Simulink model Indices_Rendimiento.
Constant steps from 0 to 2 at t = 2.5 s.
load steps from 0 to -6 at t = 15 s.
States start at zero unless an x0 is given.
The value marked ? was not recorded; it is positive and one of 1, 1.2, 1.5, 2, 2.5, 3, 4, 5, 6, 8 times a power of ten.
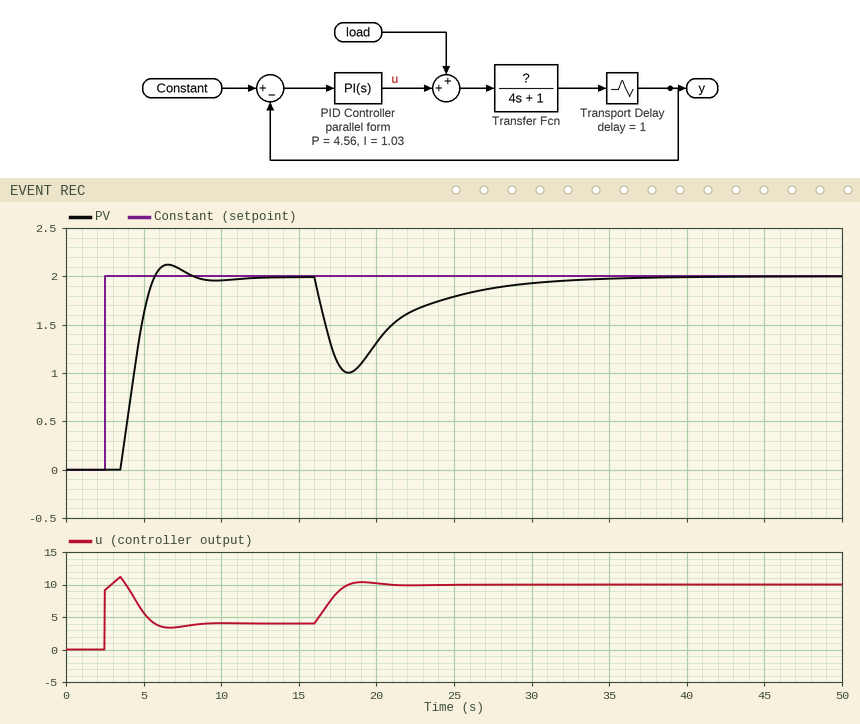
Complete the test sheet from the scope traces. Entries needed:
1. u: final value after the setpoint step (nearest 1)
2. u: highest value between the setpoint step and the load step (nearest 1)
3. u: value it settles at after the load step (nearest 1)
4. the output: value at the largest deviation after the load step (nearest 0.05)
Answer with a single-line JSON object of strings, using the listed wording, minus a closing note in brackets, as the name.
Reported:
{"u: final value after the setpoint step": "4", "u: highest value between the setpoint step and the load step": "11", "u: value it settles at after the load step": "10", "the output: value at the largest deviation after the load step": "1.00"}
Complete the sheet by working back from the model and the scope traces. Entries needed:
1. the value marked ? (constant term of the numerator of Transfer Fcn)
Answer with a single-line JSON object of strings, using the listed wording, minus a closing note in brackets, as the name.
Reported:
{"the value marked ?": "0.5"}
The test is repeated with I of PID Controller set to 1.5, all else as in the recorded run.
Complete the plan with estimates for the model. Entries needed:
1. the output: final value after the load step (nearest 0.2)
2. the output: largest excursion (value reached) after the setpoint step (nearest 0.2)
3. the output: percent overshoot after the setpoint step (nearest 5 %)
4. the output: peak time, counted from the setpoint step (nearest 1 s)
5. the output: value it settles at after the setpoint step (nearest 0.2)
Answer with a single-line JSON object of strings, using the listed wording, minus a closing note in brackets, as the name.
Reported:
{"the output: final value after the load step": "2.0", "the output: largest excursion (value reached) after the setpoint step": "2.4", "the output: percent overshoot after the setpoint step": "20 %", "the output: peak time, counted from the setpoint step": "4 s", "the output: value it settles at after the setpoint step": "2.0"}
